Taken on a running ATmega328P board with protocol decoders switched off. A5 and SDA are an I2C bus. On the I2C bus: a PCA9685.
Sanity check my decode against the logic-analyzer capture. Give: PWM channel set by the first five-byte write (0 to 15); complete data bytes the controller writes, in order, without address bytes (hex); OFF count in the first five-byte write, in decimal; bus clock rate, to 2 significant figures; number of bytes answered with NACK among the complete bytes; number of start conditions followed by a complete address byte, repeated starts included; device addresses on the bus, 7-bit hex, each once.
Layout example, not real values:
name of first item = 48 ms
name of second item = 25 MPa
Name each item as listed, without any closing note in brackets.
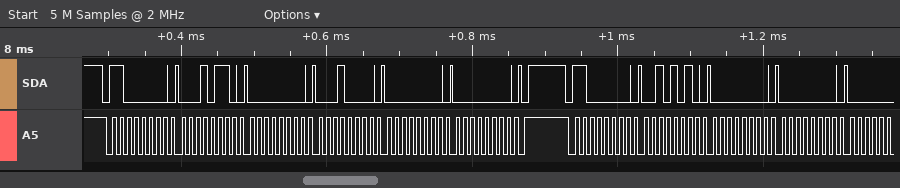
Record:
PWM channel set by the first five-byte write = 4
complete data bytes the controller writes, in order, without address bytes = 16 00 10 00 00 2A 00 00
OFF count in the first five-byte write, in decimal = 0
bus clock rate, to 2 significant figures = 100 kHz
number of bytes answered with NACK among the complete bytes = 0
number of start conditions followed by a complete address byte, repeated starts included = 2
device addresses on the bus, 7-bit hex, each once = 0x60
